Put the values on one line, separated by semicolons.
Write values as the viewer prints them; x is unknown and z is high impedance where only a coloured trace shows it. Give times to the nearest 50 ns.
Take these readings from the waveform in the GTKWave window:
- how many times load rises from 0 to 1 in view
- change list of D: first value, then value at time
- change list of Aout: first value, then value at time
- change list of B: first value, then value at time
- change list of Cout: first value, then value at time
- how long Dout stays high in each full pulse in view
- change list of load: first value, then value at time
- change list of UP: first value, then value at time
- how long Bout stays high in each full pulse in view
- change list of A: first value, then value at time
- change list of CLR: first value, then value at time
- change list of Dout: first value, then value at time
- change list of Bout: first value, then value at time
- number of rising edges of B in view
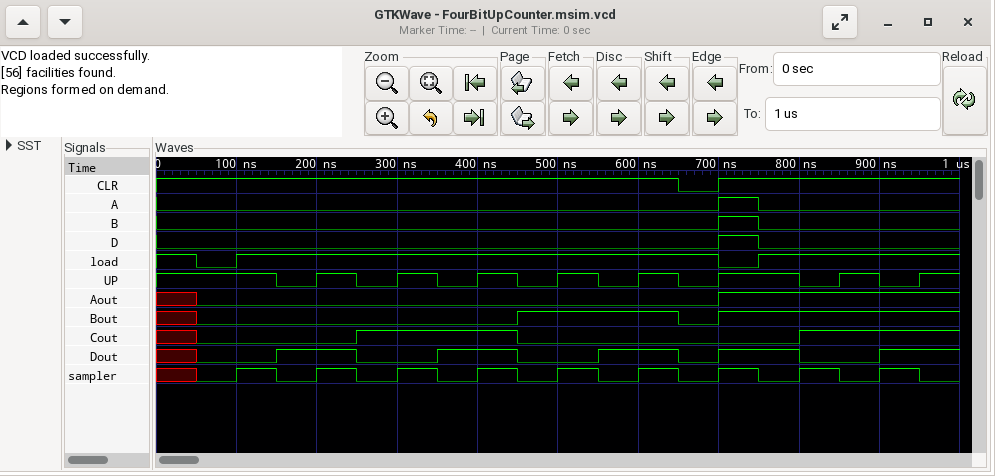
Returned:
2; 0, 1 at 700 ns, 0 at 750 ns; x, 0 at 50 ns, 1 at 700 ns; 0, 1 at 700 ns, 0 at 750 ns; x, 0 at 50 ns, 1 at 250 ns, 0 at 450 ns, 1 at 800 ns; 100 ns, 100 ns, 100 ns, 100 ns; 1, 0 at 50 ns, 1 at 100 ns, 0 at 700 ns, 1 at 750 ns; 1, 0 at 150 ns, 1 at 200 ns, 0 at 250 ns, 1 at 300 ns, 0 at 350 ns, 1 at 400 ns, 0 at 450 ns, 1 at 500 ns, 0 at 550 ns, 1 at 600 ns, 0 at 650 ns, 1 at 700 ns, 0 at 800 ns, 1 at 850 ns, 0 at 900 ns, 1 at 950 ns; 200 ns; 0, 1 at 700 ns, 0 at 750 ns; 1, 0 at 650 ns, 1 at 700 ns; x, 0 at 50 ns, 1 at 150 ns, 0 at 250 ns, 1 at 350 ns, 0 at 450 ns, 1 at 550 ns, 0 at 650 ns, 1 at 700 ns, 0 at 800 ns, 1 at 900 ns; x, 0 at 50 ns, 1 at 450 ns, 0 at 650 ns, 1 at 700 ns; 1
